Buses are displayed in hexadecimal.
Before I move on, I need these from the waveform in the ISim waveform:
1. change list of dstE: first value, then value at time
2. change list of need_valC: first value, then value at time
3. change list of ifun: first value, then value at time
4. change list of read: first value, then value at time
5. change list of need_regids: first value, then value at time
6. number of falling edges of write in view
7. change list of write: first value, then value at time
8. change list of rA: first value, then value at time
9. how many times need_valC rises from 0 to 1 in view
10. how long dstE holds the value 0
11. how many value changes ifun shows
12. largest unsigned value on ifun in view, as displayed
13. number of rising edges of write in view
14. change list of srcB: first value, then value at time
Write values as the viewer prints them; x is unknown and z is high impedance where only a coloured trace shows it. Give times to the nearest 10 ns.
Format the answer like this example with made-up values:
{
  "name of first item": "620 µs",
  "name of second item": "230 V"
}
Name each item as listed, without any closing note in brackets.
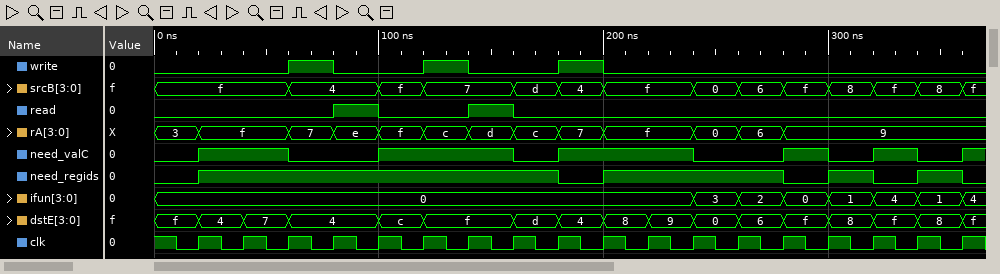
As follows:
{
  "change list of dstE: first value, then value at time": "f, 4 at 20 ns, 7 at 40 ns, 4 at 60 ns, c at 100 ns, f at 120 ns, d at 160 ns, 4 at 180 ns, 8 at 200 ns, 9 at 220 ns, 0 at 240 ns, 6 at 260 ns, f at 280 ns, 8 at 300 ns, f at 320 ns, 8 at 340 ns, f at 360 ns",
  "change list of need_valC: first value, then value at time": "0, 1 at 20 ns, 0 at 60 ns, 1 at 100 ns, 0 at 160 ns, 1 at 180 ns, 0 at 240 ns, 1 at 280 ns, 0 at 300 ns, 1 at 320 ns, 0 at 340 ns, 1 at 360 ns",
  "change list of ifun: first value, then value at time": "0, 3 at 240 ns, 2 at 260 ns, 0 at 280 ns, 1 at 300 ns, 4 at 320 ns, 1 at 340 ns, 4 at 360 ns",
  "change list of read: first value, then value at time": "0, 1 at 80 ns, 0 at 100 ns, 1 at 140 ns, 0 at 160 ns",
  "change list of need_regids: first value, then value at time": "0, 1 at 20 ns, 0 at 180 ns, 1 at 200 ns, 0 at 280 ns, 1 at 300 ns, 0 at 320 ns, 1 at 340 ns, 0 at 360 ns",
  "number of falling edges of write in view": "3",
  "change list of write: first value, then value at time": "0, 1 at 60 ns, 0 at 80 ns, 1 at 120 ns, 0 at 140 ns, 1 at 180 ns, 0 at 200 ns",
  "change list of rA: first value, then value at time": "3, f at 20 ns, 7 at 60 ns, e at 80 ns, f at 100 ns, c at 120 ns, d at 140 ns, c at 160 ns, 7 at 180 ns, f at 200 ns, 0 at 240 ns, 6 at 260 ns, 9 at 280 ns",
  "how many times need_valC rises from 0 to 1 in view": "6",
  "how long dstE holds the value 0": "20 ns",
  "how many value changes ifun shows": "7",
  "largest unsigned value on ifun in view, as displayed": "4",
  "number of rising edges of write in view": "3",
  "change list of srcB: first value, then value at time": "f, 4 at 60 ns, f at 100 ns, 7 at 120 ns, d at 160 ns, 4 at 180 ns, f at 200 ns, 0 at 240 ns, 6 at 260 ns, f at 280 ns, 8 at 300 ns, f at 320 ns, 8 at 340 ns, f at 360 ns"
}
